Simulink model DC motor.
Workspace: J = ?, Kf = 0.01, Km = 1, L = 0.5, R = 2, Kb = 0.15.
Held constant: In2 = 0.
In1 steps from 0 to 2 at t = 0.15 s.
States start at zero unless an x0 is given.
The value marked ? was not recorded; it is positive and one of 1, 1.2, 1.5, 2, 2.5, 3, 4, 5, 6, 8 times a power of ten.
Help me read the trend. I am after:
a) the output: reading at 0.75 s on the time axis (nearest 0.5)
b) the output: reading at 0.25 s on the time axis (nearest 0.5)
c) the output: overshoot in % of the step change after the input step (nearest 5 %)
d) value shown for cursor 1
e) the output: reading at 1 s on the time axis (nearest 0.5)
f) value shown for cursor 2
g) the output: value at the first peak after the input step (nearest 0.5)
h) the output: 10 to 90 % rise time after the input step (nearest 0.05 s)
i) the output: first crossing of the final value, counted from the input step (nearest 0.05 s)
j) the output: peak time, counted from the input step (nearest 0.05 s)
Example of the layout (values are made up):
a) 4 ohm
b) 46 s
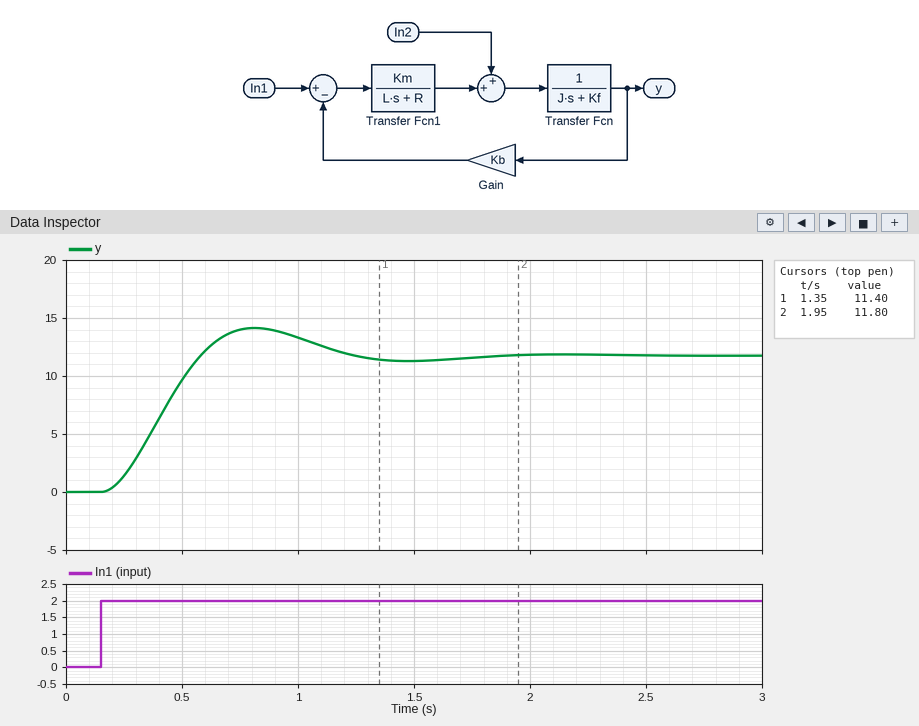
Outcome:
a) 14.0
b) 1.5
c) 20 %
d) 11.40
e) 13.5
f) 11.80
g) 14.0
h) 0.30 s
i) 0.45 s
j) 0.65 s
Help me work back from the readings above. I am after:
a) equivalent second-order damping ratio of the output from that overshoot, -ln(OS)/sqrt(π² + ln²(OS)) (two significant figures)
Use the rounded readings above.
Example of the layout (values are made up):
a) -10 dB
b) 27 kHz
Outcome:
a) 0.46
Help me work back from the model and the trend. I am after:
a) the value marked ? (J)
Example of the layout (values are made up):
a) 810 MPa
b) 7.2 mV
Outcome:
a) 0.012
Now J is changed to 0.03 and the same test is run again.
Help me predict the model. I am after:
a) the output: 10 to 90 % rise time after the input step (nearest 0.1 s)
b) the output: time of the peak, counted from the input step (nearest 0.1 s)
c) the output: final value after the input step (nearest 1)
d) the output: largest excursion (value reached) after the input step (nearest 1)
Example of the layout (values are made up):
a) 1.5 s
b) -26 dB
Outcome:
a) 0.6 s
b) 1.2 s
c) 12
d) 13
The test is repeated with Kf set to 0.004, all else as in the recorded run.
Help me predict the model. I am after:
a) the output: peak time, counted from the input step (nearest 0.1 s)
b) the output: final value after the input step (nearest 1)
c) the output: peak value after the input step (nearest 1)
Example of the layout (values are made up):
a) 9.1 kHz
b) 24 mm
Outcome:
a) 0.7 s
b) 13
c) 16
